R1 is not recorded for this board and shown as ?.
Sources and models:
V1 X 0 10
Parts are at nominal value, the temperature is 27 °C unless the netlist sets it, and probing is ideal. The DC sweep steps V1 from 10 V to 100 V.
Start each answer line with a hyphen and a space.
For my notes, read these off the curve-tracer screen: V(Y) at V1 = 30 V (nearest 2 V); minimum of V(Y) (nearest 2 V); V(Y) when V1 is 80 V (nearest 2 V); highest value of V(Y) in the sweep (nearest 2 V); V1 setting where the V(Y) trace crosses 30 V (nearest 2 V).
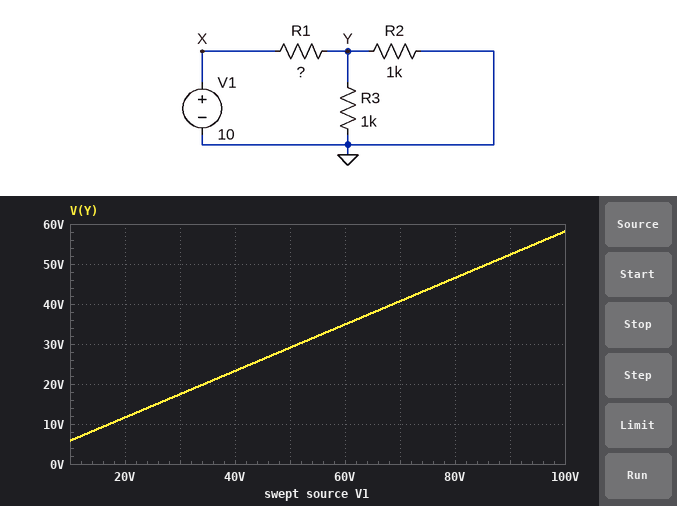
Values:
- 18 V
- 6 V
- 46 V
- 58 V
- 52 V
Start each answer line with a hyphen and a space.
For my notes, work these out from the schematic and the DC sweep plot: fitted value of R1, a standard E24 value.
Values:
- 360 Ω
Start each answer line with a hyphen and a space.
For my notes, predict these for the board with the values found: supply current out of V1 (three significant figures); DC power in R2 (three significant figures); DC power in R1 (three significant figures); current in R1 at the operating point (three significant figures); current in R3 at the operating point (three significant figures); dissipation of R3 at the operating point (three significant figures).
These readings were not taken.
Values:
- 11.6 mA
- 33.8 mW
- 48.7 mW
- 11.6 mA
- 5.81 mA
- 33.8 mW
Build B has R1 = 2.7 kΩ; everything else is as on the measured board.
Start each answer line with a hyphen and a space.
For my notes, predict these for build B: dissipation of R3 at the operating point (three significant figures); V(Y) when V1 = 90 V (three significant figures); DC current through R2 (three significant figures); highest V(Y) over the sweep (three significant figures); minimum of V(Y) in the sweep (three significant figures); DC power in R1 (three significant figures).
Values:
- 2.44 mW
- 14.1 V
- 1.56 mA
- 15.6 V
- 1.56 V
- 26.4 mW
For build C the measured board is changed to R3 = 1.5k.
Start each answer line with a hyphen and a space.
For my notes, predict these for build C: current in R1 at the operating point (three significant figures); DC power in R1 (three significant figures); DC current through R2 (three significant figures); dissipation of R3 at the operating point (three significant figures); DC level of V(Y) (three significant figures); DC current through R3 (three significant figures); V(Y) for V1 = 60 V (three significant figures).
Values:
- 10.4 mA
- 39.1 mW
- 6.25 mA
- 26.0 mW
- 6.25 V
- 4.17 mA
- 37.5 V
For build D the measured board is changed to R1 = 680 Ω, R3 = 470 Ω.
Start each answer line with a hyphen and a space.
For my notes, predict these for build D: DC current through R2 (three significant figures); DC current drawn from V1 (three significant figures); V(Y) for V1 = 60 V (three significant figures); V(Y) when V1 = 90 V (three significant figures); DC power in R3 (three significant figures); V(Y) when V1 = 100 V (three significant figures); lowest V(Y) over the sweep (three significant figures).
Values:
- 3.20 mA
- 10.0 mA
- 19.2 V
- 28.8 V
- 21.8 mW
- 32.0 V
- 3.20 V
